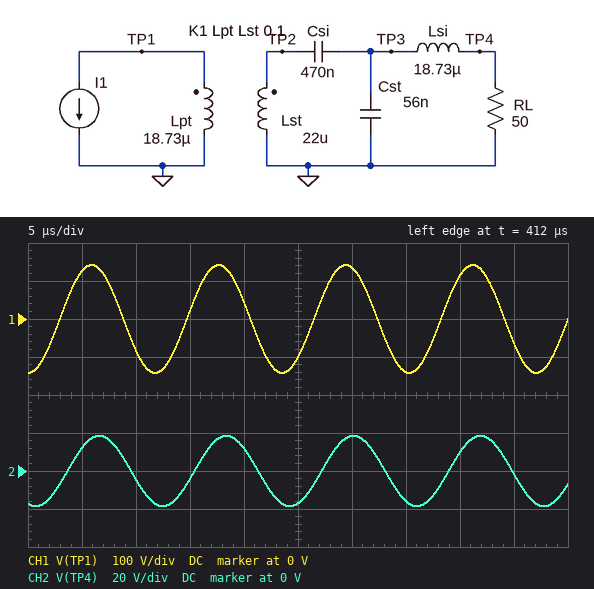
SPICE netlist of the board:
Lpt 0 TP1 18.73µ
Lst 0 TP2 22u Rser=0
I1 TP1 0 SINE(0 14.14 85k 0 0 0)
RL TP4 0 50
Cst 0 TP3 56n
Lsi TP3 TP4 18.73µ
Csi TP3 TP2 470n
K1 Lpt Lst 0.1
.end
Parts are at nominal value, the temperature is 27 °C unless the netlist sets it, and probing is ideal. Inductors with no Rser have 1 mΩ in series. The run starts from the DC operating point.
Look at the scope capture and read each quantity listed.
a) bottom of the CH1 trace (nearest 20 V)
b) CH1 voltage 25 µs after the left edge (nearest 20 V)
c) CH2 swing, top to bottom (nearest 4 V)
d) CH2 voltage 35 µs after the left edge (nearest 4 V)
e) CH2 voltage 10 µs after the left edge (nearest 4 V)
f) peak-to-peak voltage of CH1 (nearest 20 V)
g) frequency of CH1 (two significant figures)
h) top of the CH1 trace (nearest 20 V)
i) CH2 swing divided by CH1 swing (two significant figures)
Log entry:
-140 V
-100 V
36 V
-16 V
-4 V
280 V
85 kHz
140 V
0.13
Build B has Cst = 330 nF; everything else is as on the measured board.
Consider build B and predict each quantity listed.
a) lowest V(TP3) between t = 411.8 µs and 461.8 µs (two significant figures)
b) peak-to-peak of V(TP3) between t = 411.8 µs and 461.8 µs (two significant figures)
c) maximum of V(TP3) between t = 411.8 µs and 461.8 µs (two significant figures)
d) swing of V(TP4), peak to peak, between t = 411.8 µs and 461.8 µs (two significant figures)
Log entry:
-41 V
83 V
41 V
81 V
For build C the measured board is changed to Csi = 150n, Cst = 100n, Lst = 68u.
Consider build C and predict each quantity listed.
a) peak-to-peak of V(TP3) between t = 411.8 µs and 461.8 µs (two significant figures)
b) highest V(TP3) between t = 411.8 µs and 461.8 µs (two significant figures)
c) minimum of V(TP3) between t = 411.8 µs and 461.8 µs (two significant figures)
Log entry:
110 V
55 V
-55 V
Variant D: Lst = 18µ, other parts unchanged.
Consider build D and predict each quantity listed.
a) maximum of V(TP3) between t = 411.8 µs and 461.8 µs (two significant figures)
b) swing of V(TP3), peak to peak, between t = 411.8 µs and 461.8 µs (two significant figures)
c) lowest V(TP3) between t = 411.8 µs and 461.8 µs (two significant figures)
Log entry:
16 V
32 V
-16 V
